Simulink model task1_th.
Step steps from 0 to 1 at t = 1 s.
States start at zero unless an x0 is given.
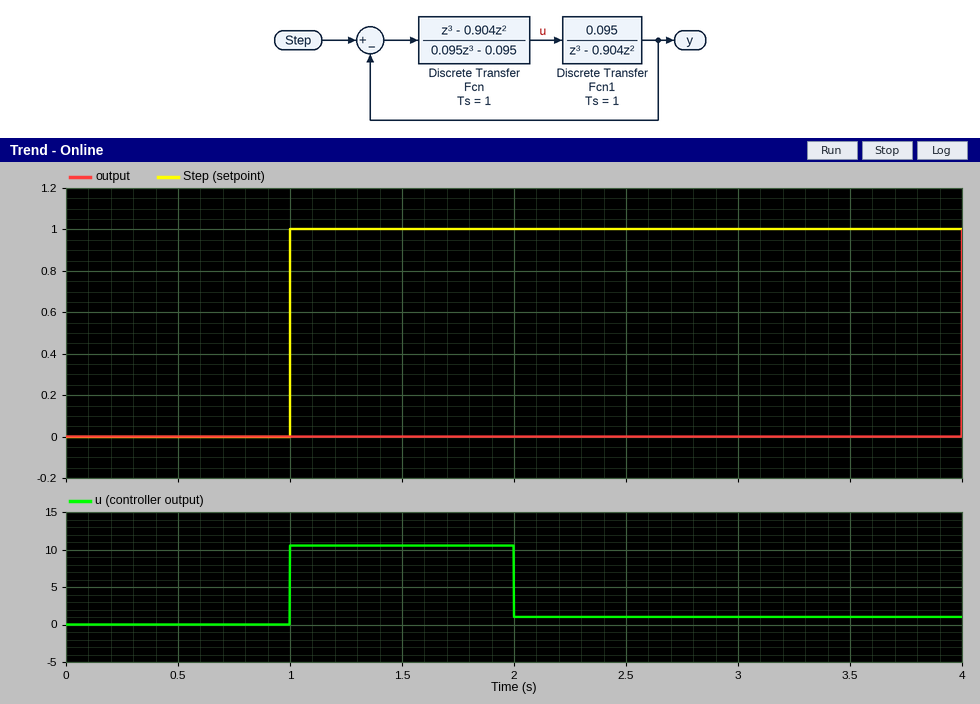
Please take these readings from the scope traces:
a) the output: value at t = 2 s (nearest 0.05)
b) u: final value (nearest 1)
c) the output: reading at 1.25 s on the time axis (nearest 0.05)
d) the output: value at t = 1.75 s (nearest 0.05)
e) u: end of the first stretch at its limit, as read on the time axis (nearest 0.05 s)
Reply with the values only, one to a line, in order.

0.00
1
0.00
0.00
2.00 s
